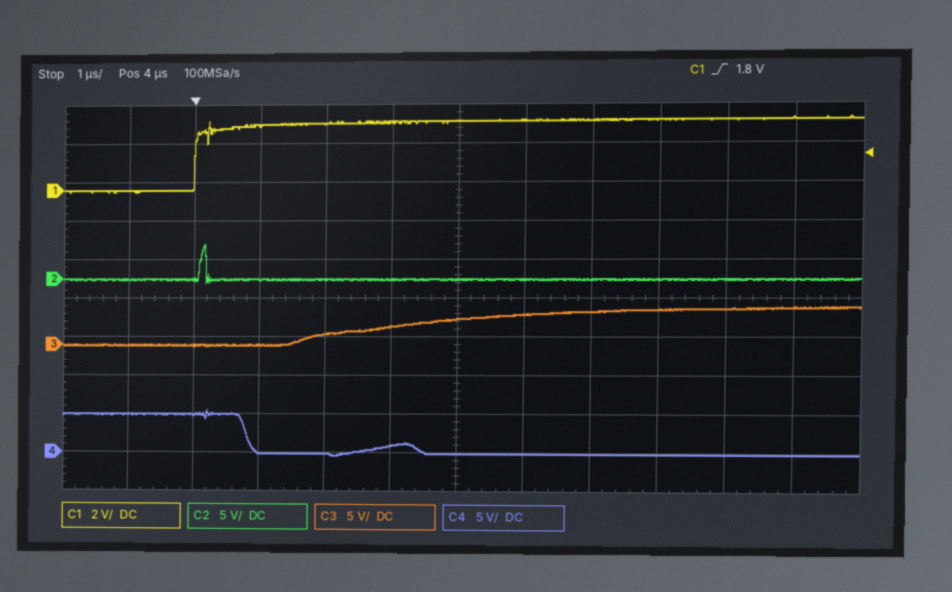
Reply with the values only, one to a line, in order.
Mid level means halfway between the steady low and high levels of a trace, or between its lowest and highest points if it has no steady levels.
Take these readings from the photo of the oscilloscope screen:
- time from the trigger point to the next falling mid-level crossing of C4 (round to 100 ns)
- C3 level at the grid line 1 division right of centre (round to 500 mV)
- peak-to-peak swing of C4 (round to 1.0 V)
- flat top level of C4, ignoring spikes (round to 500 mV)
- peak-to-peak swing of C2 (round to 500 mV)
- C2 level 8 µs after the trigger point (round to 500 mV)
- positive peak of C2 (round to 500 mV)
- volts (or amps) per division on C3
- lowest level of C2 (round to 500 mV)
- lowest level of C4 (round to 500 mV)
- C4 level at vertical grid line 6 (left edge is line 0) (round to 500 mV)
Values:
800 ns
4.0 V
6.0 V
5.0 V
5.0 V
0.0 V
4.5 V
5 V
-500 mV
-500 mV
0.0 V
